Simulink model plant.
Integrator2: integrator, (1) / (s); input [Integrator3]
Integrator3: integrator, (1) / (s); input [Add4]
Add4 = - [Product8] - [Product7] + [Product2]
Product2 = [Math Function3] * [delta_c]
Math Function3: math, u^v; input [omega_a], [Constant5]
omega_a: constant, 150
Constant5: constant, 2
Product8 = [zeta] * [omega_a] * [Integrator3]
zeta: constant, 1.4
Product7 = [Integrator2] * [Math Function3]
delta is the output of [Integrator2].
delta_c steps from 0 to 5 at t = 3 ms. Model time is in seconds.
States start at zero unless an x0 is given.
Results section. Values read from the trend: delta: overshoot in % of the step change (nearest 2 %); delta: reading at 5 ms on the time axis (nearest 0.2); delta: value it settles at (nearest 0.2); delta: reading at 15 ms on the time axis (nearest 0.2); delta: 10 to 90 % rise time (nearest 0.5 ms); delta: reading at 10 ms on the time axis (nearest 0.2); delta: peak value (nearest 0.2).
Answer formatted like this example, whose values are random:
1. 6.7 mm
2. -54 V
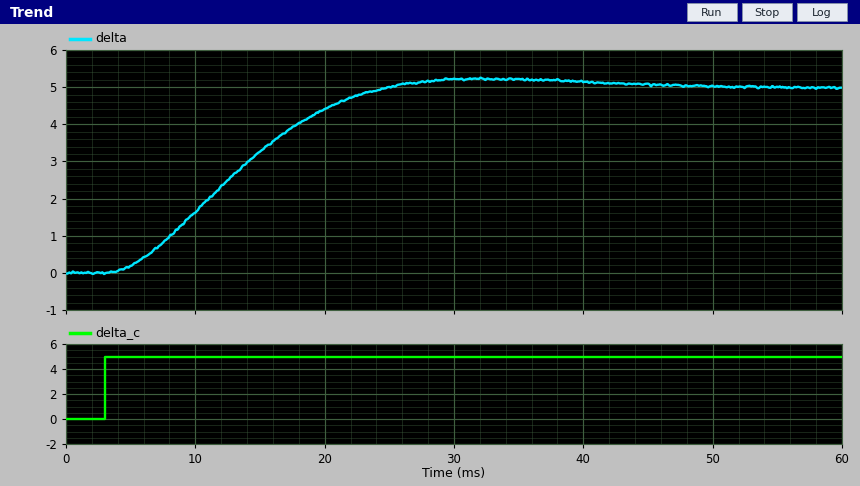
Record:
1. 4 %
2. 0.2
3. 5.0
4. 3.2
5. 14.0 ms
6. 1.6
7. 5.2
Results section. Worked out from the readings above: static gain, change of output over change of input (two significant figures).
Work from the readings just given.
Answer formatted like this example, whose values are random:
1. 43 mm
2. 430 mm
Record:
1. 1.0
